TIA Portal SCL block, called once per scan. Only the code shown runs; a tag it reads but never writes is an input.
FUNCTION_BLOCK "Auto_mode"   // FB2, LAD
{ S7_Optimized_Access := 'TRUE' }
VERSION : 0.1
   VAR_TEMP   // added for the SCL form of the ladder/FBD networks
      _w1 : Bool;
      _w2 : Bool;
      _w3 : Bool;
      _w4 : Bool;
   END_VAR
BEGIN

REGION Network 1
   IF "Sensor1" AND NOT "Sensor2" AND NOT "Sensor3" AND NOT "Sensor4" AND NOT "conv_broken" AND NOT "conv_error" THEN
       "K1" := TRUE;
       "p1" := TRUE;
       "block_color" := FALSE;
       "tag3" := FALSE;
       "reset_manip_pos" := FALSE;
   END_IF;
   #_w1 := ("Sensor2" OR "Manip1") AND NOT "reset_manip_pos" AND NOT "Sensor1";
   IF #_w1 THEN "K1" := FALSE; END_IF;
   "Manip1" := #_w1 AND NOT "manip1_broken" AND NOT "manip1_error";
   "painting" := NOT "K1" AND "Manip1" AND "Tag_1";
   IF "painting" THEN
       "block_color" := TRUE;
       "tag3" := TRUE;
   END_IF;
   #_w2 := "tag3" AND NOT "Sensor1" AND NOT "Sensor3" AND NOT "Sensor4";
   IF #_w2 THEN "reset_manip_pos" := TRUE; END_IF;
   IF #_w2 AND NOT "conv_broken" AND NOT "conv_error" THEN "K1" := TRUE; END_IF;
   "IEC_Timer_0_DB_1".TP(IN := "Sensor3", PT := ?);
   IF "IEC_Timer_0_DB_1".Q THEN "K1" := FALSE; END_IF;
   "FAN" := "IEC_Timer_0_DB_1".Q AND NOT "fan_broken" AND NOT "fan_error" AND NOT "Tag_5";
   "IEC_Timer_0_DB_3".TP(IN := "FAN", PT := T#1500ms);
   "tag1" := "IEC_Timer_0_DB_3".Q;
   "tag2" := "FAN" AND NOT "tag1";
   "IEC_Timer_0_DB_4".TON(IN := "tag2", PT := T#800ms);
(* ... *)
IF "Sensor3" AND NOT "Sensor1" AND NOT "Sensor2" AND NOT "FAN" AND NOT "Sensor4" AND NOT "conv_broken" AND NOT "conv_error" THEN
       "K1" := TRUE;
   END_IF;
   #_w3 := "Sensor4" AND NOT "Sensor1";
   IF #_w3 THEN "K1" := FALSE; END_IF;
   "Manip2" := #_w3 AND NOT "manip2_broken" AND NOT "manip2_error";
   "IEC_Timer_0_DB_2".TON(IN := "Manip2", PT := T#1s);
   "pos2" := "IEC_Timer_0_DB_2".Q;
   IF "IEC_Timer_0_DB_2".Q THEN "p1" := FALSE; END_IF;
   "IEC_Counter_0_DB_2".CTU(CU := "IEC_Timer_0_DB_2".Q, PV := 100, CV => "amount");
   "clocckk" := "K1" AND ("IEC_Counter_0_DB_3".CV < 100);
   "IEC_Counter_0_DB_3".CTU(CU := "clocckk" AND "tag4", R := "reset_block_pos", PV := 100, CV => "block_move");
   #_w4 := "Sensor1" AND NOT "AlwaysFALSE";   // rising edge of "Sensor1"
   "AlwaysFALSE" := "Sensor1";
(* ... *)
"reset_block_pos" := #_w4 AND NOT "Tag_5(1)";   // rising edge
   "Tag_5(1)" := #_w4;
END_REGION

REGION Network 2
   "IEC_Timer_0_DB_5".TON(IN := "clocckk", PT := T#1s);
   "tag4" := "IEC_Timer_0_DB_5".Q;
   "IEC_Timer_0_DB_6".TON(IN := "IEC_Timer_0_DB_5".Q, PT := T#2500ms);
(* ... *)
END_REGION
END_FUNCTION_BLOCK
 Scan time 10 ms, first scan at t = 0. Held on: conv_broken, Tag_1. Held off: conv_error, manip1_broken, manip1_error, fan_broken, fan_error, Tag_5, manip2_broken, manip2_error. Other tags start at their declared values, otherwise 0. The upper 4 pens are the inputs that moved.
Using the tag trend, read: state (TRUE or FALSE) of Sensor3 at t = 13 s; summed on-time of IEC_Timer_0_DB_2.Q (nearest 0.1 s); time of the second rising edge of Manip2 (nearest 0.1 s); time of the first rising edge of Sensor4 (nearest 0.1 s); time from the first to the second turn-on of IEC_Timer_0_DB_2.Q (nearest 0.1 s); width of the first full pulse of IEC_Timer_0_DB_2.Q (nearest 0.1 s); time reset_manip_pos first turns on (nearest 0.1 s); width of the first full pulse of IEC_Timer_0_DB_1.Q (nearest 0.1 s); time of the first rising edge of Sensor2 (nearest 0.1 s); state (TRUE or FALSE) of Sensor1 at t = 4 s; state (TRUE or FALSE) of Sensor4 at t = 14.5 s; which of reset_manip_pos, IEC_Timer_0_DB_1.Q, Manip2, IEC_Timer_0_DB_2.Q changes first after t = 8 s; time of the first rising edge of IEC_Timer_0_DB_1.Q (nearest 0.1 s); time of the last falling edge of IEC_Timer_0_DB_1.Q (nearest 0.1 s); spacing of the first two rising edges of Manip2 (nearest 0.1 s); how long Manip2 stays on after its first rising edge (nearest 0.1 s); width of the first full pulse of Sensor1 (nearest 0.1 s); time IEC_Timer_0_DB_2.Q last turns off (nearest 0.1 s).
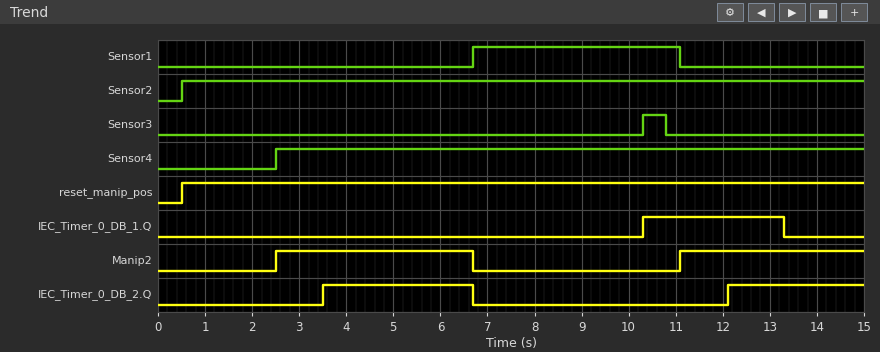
FALSE
6.1 s
11.1 s
2.5 s
8.6 s
3.2 s
0.5 s
3.0 s
0.5 s
FALSE
TRUE
IEC_Timer_0_DB_1.Q
10.3 s
13.3 s
8.6 s
4.2 s
4.4 s
6.7 s
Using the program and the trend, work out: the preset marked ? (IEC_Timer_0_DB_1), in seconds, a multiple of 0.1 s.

3.0 s
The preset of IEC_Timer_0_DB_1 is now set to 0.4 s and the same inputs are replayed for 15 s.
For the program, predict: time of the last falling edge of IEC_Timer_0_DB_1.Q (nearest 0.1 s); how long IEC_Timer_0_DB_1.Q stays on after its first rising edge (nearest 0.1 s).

10.7 s
0.4 s
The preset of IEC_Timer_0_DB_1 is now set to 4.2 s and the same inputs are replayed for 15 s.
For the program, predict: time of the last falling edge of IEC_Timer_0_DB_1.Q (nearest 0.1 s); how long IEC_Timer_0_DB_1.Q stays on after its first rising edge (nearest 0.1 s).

14.5 s
4.2 s
